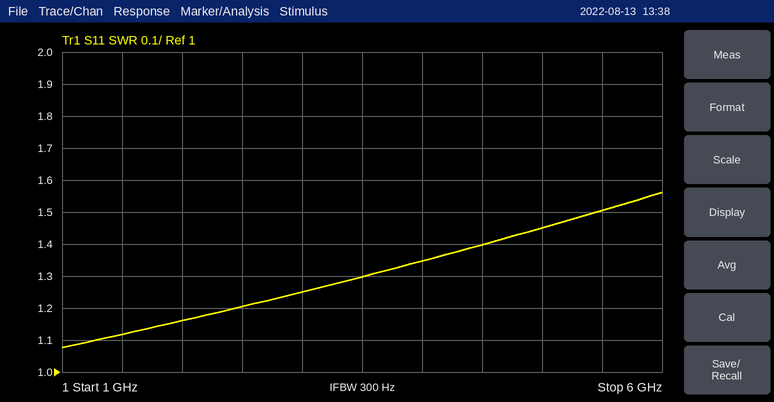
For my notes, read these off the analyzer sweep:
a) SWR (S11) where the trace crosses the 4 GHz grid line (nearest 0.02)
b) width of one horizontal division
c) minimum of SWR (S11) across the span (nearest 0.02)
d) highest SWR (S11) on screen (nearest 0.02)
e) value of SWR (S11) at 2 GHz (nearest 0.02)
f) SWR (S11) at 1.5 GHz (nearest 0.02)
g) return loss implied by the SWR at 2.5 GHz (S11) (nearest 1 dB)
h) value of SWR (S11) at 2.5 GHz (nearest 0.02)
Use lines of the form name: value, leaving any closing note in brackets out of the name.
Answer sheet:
SWR (S11) where the trace crosses the 4 GHz grid line: 1.34
width of one horizontal division: 500 MHz
minimum of SWR (S11) across the span: 1.08
highest SWR (S11) on screen: 1.56
value of SWR (S11) at 2 GHz: 1.16
SWR (S11) at 1.5 GHz: 1.12
return loss implied by the SWR at 2.5 GHz (S11): 21 dB
value of SWR (S11) at 2.5 GHz: 1.20
